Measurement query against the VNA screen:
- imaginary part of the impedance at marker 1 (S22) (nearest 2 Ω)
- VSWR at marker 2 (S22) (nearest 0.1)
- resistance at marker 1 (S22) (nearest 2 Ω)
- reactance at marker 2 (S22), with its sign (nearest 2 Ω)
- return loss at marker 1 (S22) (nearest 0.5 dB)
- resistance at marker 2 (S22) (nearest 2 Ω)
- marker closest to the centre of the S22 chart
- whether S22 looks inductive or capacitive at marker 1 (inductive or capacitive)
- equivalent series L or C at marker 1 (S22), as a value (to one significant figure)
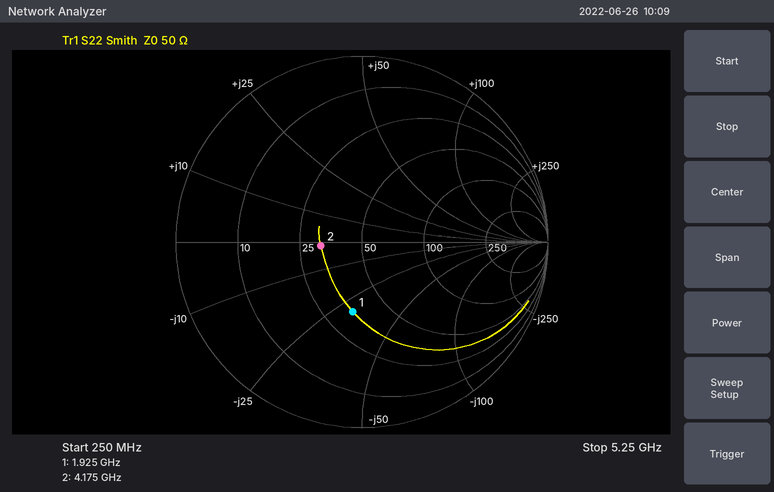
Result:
-30 Ω
1.6
34 Ω
-2 Ω
8.5 dB
32 Ω
marker 2
capacitive
3 pF
